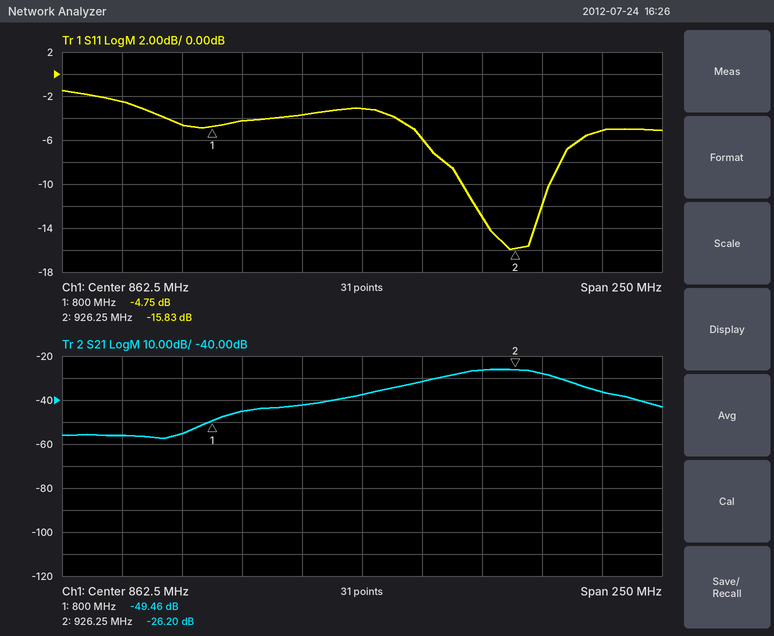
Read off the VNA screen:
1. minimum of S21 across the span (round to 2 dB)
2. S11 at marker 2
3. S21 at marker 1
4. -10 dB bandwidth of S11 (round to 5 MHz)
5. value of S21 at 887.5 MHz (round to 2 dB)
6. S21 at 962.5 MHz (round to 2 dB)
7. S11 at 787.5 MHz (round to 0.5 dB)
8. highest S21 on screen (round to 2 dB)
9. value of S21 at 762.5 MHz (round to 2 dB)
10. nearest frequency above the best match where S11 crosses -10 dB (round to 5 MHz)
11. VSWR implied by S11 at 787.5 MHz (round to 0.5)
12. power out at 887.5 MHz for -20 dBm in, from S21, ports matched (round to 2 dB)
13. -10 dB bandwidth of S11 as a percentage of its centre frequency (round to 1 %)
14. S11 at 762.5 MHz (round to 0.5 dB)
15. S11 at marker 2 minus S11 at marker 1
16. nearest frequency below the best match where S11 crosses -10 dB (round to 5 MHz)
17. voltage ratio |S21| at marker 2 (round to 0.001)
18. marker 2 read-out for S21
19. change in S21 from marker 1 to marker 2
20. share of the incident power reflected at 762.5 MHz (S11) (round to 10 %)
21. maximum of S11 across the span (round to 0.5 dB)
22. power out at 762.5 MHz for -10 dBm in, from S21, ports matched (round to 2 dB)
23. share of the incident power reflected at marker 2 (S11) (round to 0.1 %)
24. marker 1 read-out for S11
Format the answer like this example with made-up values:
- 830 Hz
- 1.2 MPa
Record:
- -58 dB
- -15.83 dB
- -49.46 dB
- 35 MHz
- -32 dB
- -36 dB
- -4.5 dB
- -26 dB
- -56 dB
- 940 MHz
- 4.0
- -52 dBm
- 4 %
- -2.5 dB
- -11.08 dB
- 905 MHz
- 0.049
- -26.20 dB
- 23.26 dB
- 60 %
- -1.5 dB
- -66 dBm
- 2.6 %
- -4.75 dB
